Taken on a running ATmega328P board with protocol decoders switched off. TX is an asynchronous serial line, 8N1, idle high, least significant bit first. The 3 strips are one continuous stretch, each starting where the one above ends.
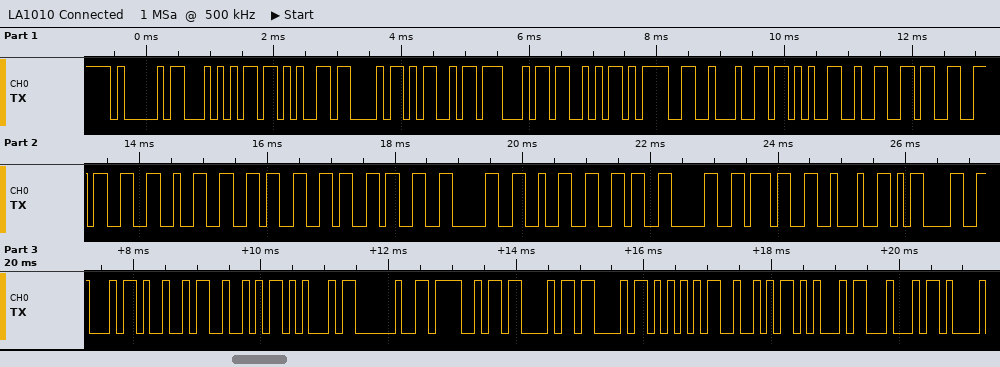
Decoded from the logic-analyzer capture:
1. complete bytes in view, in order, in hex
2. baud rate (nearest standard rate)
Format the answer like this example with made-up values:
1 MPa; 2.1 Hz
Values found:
41 54 2B 43 4D 47 53 3D 22 2B 32 33 33 32 36 36 33 30 32 36 30 37 22 0D 46 49 52 45 20 4F 43 43 55 52 45 44; 9600 baud
